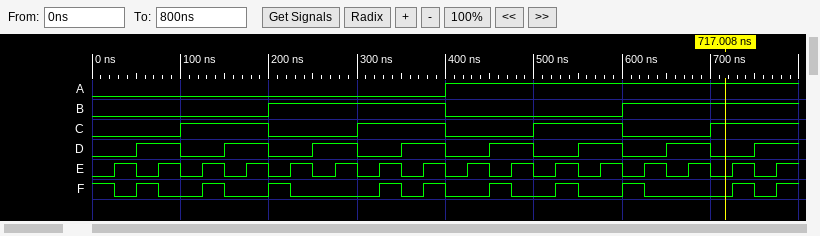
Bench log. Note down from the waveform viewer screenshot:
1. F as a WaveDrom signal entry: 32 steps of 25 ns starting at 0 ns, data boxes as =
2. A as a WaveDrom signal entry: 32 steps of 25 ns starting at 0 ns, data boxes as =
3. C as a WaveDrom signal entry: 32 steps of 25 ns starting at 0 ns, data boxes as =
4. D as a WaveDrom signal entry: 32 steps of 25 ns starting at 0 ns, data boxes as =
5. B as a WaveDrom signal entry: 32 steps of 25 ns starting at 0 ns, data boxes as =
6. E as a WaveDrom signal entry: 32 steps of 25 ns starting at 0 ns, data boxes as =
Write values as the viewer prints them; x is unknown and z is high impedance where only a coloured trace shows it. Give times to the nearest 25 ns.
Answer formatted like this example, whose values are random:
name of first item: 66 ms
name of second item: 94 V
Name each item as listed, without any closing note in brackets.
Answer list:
F as a WaveDrom signal entry: 32 steps of 25 ns starting at 0 ns, data boxes as =: {name: 'F', wave: '1010.10.10...1010.10.10.10...101'}
A as a WaveDrom signal entry: 32 steps of 25 ns starting at 0 ns, data boxes as =: {name: 'A', wave: '0...............1...............'}
C as a WaveDrom signal entry: 32 steps of 25 ns starting at 0 ns, data boxes as =: {name: 'C', wave: '0...1...0...1...0...1...0...1...'}
D as a WaveDrom signal entry: 32 steps of 25 ns starting at 0 ns, data boxes as =: {name: 'D', wave: '0.1.0.1.0.1.0.1.0.1.0.1.0.1.0.1.'}
B as a WaveDrom signal entry: 32 steps of 25 ns starting at 0 ns, data boxes as =: {name: 'B', wave: '0.......1.......0.......1.......'}
E as a WaveDrom signal entry: 32 steps of 25 ns starting at 0 ns, data boxes as =: {name: 'E', wave: '01010101010101010101010101010101'}
